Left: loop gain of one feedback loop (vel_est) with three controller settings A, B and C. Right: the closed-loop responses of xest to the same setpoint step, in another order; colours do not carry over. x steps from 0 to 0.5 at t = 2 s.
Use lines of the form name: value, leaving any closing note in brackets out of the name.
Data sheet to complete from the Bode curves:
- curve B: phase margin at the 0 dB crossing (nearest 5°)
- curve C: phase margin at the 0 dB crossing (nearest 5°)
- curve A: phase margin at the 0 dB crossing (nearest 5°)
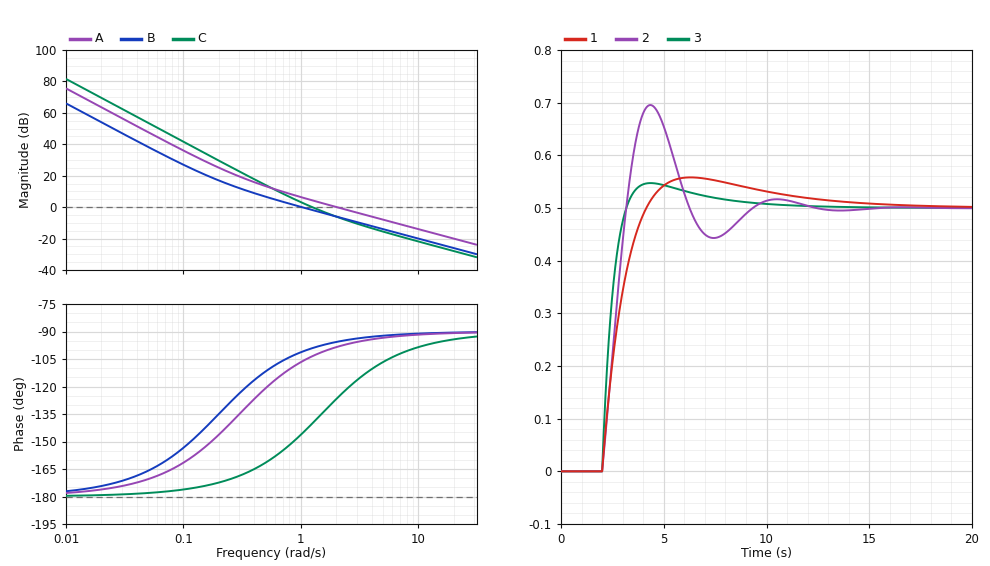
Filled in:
curve B: phase margin at the 0 dB crossing: 80°
curve C: phase margin at the 0 dB crossing: 40°
curve A: phase margin at the 0 dB crossing: 80°
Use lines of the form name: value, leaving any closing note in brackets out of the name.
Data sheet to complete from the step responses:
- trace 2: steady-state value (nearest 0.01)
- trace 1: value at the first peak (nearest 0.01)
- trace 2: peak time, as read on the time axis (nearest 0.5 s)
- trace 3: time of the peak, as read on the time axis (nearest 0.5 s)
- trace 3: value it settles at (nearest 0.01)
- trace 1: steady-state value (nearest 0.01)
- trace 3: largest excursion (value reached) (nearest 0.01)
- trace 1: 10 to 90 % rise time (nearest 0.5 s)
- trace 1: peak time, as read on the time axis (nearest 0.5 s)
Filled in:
trace 2: steady-state value: 0.50
trace 1: value at the first peak: 0.56
trace 2: peak time, as read on the time axis: 4.5 s
trace 3: time of the peak, as read on the time axis: 4.5 s
trace 3: value it settles at: 0.50
trace 1: steady-state value: 0.50
trace 3: largest excursion (value reached): 0.55
trace 1: 10 to 90 % rise time: 1.5 s
trace 1: peak time, as read on the time axis: 6.5 s
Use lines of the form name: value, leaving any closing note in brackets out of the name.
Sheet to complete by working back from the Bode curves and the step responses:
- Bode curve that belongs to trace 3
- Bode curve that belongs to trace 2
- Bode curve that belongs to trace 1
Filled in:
Bode curve that belongs to trace 3: A
Bode curve that belongs to trace 2: C
Bode curve that belongs to trace 1: B
